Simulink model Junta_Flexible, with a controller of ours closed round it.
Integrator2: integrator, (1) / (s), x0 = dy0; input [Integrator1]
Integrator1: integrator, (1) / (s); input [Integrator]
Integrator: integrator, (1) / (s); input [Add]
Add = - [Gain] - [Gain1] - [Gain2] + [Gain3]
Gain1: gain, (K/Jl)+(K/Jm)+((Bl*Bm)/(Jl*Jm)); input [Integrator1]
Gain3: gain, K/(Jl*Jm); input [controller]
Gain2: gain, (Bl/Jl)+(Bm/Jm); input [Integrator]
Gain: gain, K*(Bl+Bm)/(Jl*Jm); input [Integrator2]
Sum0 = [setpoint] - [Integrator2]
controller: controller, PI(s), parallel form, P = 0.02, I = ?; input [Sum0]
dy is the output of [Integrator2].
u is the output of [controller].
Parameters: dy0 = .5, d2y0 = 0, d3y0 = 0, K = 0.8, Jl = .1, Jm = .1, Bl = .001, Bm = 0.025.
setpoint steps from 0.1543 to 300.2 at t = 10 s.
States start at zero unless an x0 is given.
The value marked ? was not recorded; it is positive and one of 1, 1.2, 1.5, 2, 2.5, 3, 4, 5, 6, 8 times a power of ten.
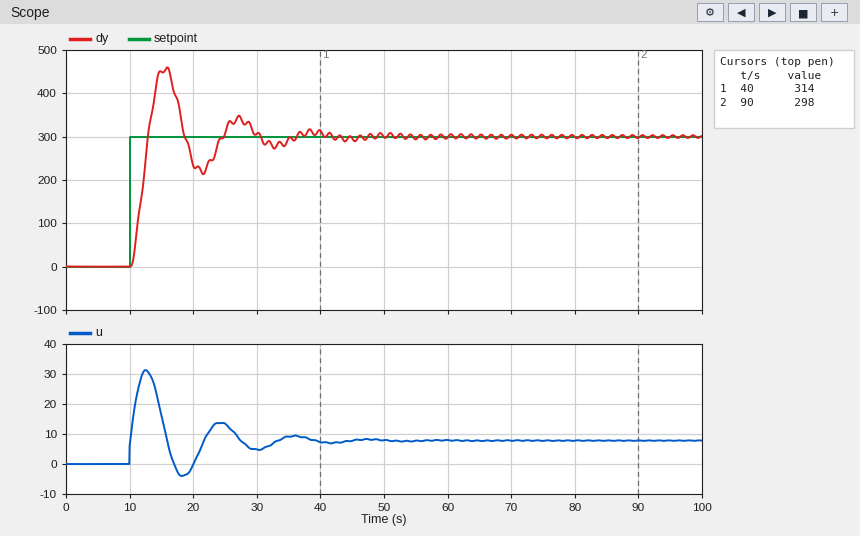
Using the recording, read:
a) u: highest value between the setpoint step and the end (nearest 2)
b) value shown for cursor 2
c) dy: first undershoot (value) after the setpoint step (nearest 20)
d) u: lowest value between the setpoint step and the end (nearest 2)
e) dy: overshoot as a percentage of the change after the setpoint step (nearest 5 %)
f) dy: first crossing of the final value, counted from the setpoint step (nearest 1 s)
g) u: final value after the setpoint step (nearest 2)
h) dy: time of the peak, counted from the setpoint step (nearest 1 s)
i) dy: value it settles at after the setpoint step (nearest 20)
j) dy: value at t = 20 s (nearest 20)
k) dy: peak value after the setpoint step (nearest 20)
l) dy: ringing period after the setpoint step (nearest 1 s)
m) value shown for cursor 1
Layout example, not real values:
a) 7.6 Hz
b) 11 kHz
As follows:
a) 32
b) 298
c) 220
d) -4
e) 55 %
f) 3 s
g) 8
h) 6 s
i) 300
j) 240
k) 460
l) 11 s
m) 314
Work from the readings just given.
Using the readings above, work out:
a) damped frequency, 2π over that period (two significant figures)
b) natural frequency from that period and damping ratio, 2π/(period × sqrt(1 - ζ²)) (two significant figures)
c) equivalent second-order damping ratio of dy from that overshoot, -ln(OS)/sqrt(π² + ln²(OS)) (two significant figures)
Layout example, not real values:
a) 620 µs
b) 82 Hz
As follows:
a) 0.57 rad/s
b) 0.58 rad/s
c) 0.19
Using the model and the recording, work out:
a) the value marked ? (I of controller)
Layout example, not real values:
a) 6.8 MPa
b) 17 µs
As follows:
a) 0.06
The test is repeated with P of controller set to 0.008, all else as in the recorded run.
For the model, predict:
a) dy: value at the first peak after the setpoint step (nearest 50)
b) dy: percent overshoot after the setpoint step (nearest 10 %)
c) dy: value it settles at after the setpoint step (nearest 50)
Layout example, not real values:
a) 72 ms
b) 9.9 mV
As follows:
a) 500
b) 60 %
c) 300
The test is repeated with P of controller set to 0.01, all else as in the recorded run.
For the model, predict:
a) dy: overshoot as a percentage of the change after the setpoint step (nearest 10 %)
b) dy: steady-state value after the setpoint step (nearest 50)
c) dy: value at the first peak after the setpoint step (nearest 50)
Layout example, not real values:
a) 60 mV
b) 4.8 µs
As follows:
a) 60 %
b) 300
c) 500
